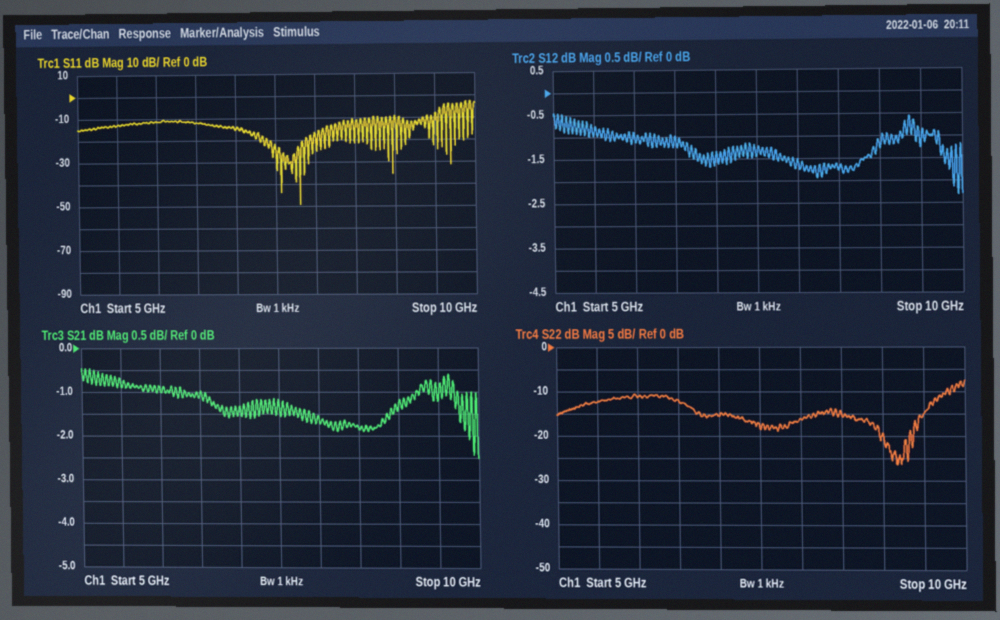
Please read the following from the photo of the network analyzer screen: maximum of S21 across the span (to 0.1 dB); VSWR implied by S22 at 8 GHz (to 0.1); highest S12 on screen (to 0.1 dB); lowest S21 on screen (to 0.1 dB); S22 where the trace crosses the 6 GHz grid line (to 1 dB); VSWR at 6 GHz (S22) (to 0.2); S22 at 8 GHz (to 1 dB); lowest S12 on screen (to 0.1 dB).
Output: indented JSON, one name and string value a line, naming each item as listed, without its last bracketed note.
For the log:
{
  "maximum of S21 across the span": "-0.5 dB",
  "VSWR implied by S22 at 8 GHz": "1.4",
  "highest S12 on screen": "-0.5 dB",
  "lowest S21 on screen": "-2.5 dB",
  "S22 where the trace crosses the 6 GHz grid line": "-11 dB",
  "VSWR at 6 GHz (S22)": "1.8",
  "S22 at 8 GHz": "-16 dB",
  "lowest S12 on screen": "-2.3 dB"
}
